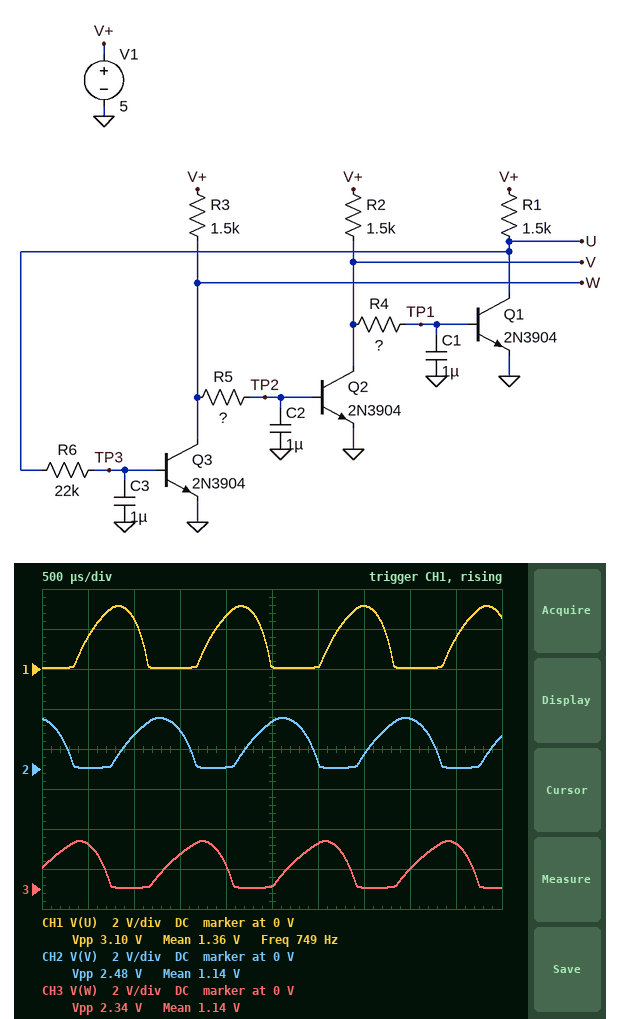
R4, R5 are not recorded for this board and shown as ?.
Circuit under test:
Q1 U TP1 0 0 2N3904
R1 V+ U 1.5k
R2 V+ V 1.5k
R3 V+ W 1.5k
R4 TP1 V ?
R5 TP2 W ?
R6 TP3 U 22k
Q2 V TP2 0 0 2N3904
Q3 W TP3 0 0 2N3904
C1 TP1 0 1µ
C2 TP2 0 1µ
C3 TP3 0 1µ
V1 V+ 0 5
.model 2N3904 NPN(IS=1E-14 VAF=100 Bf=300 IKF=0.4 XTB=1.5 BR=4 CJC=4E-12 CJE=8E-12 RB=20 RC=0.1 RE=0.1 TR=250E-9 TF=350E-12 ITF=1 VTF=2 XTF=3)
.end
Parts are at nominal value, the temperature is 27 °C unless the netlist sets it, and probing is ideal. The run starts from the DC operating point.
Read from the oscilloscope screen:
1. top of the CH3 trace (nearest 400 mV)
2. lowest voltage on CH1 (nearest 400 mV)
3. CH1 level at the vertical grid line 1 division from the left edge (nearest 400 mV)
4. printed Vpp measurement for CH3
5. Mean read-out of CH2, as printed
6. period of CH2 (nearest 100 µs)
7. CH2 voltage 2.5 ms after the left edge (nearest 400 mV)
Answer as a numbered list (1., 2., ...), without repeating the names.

1. 2.4 V
2. 0 V
3. 1.6 V
4. 2.34 V
5. 1.14 V
6. 1.3 ms
7. 2.4 V
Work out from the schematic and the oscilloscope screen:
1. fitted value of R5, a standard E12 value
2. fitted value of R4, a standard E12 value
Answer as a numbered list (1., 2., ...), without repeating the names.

1. 15 kΩ
2. 10 kΩ
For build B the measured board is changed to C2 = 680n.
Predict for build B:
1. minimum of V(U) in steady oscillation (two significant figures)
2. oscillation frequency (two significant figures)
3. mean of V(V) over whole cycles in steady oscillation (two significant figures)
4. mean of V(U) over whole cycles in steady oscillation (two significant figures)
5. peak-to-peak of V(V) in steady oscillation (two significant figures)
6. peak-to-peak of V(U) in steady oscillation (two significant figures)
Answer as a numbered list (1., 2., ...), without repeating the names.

1. 46 mV
2. 840 Hz
3. 1.3 V
4. 1.2 V
5. 2.8 V
6. 3.0 V
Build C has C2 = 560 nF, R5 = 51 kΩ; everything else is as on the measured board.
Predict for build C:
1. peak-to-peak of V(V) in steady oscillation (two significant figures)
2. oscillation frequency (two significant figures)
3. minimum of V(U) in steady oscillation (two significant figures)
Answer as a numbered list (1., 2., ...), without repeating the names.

1. 2.2 V
2. 630 Hz
3. 51 mV
